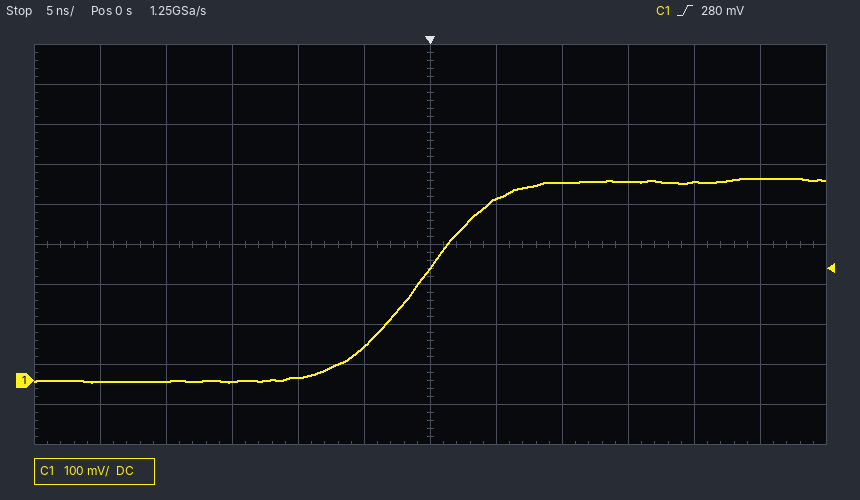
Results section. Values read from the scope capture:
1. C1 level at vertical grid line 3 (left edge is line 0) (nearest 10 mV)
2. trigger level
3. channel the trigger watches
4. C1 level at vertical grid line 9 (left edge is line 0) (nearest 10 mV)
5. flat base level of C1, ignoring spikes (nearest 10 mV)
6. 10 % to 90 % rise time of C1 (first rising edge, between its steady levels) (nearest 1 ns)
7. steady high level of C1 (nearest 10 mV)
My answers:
0 mV
280 mV
C1
500 mV
0 mV
11 ns
500 mV
